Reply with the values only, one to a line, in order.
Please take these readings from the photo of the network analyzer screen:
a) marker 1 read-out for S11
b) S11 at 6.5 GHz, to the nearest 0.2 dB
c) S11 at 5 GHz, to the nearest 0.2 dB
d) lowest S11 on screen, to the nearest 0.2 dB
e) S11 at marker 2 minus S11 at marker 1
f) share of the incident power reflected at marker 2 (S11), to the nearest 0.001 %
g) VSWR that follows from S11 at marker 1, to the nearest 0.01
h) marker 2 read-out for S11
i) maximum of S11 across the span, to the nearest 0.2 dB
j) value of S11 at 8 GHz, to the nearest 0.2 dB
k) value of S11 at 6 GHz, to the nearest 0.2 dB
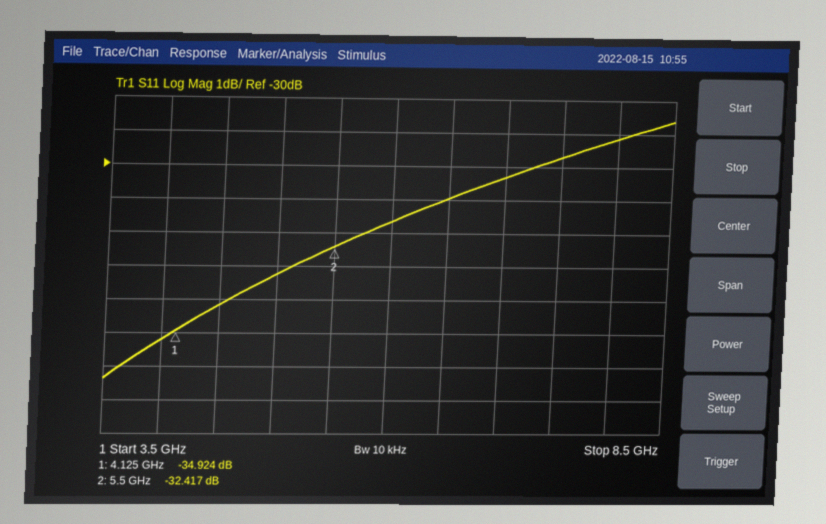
-34.924 dB
-31.0 dB
-33.2 dB
-36.4 dB
2.507 dB
0.057 %
1.04
-32.417 dB
-28.6 dB
-29.2 dB
-31.6 dB
